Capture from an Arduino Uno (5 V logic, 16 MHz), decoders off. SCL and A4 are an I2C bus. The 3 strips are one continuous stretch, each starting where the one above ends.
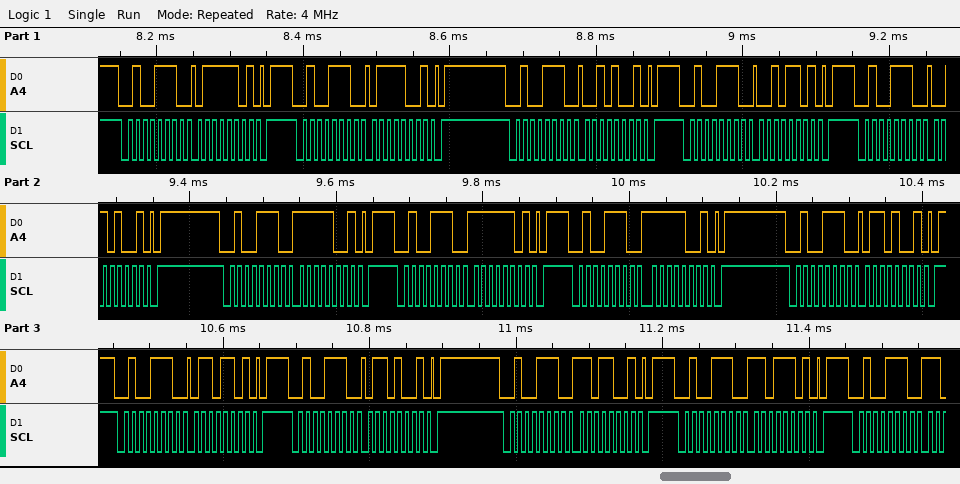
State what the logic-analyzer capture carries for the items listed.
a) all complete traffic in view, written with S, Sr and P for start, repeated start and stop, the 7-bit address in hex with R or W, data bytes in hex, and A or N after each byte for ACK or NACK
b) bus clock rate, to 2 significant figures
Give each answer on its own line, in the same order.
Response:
S 27W A 7D A P S 27W A 79 A P S 27W A 29 A P S 27W A 2D A P S 27W A 29 A P S 27W A F9 A P S 27W A FD A P S 27W A F9 A P S 27W A 69 A P S 27W A 6D A P S 27W A 69 A P S 27W A D9 A P S 27W A DD A P S 27W A
100 kHz
